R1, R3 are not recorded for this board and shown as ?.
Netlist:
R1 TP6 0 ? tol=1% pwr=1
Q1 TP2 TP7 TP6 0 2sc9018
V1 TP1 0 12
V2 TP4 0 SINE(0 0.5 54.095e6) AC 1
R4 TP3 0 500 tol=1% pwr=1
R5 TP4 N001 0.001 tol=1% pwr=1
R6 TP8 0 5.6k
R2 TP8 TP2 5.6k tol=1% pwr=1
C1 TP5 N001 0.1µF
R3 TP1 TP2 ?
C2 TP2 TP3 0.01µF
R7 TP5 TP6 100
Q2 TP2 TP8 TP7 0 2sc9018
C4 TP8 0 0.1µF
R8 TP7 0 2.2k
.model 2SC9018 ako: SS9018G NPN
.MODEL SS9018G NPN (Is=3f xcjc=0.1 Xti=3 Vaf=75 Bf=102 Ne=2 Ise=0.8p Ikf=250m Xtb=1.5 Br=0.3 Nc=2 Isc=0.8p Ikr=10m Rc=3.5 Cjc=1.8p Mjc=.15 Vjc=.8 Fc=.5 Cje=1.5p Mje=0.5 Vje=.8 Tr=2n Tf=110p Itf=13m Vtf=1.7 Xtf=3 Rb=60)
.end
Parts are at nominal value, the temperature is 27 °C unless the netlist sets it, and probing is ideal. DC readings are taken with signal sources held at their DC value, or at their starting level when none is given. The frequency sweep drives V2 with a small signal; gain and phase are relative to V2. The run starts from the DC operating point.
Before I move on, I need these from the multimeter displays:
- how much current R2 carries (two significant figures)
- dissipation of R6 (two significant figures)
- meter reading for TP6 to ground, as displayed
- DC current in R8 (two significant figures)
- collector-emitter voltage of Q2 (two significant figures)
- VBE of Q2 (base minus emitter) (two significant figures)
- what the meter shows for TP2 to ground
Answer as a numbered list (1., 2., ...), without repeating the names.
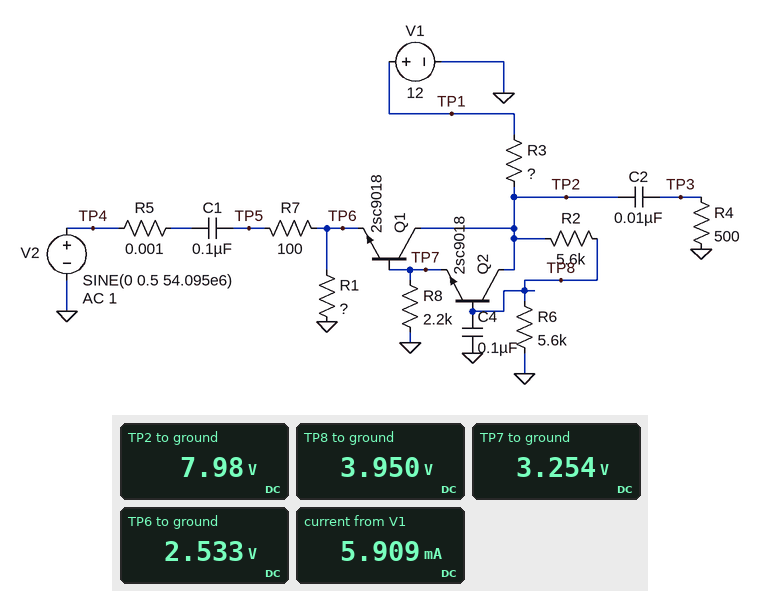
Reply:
1. 720 µA
2. 2.8 mW
3. 2.533 V
4. 1.5 mA
5. 4.7 V
6. 700 mV
7. 7.98 V
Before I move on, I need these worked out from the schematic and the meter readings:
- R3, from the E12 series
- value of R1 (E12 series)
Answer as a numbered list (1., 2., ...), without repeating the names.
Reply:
1. 680 Ω
2. 680 Ω
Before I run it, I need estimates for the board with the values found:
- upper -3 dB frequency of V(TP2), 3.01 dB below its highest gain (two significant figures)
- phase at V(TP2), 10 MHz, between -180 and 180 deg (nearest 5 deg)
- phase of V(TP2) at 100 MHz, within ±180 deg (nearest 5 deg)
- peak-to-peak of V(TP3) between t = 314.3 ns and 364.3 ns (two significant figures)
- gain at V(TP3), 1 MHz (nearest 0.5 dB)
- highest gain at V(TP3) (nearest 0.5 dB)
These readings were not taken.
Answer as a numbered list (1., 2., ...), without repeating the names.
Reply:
1. 230 MHz
2. 0 deg
3. -20 deg
4. 2.3 V
5. 8.0 dB
6. 8.0 dB
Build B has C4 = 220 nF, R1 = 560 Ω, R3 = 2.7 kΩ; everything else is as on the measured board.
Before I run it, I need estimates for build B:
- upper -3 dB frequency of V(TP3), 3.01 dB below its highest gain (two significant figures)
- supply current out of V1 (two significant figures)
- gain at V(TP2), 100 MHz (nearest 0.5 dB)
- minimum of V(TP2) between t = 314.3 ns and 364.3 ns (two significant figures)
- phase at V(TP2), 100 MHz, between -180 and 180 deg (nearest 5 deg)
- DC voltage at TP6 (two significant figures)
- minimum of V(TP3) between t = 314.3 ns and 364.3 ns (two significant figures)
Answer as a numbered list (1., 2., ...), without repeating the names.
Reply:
1. 190 MHz
2. 2.7 mA
3. 9.5 dB
4. 2.9 V
5. -35 deg
6. 900 mV
7. -1.7 V
